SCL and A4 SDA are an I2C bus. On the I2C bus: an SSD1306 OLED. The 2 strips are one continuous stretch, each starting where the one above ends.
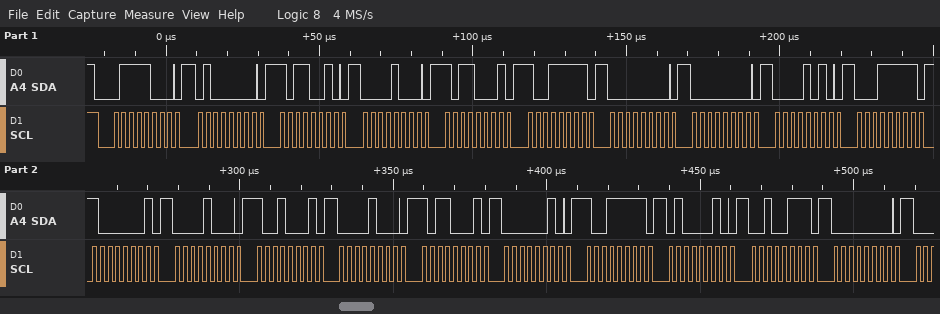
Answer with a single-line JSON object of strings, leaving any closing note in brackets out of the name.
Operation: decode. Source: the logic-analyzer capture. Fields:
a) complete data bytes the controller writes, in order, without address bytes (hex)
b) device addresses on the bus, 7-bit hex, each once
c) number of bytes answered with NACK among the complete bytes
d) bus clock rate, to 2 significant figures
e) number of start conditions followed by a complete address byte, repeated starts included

{"complete data bytes the controller writes, in order, without address bytes": "40 B2 08 B1 9F 00 00 0A 1F 81 08 91 08 B1 02 9F 42 27 00", "device addresses on the bus, 7-bit hex, each once": "0x3C", "number of bytes answered with NACK among the complete bytes": "0", "bus clock rate, to 2 significant figures": "400 kHz", "number of start conditions followed by a complete address byte, repeated starts included": "1"}
